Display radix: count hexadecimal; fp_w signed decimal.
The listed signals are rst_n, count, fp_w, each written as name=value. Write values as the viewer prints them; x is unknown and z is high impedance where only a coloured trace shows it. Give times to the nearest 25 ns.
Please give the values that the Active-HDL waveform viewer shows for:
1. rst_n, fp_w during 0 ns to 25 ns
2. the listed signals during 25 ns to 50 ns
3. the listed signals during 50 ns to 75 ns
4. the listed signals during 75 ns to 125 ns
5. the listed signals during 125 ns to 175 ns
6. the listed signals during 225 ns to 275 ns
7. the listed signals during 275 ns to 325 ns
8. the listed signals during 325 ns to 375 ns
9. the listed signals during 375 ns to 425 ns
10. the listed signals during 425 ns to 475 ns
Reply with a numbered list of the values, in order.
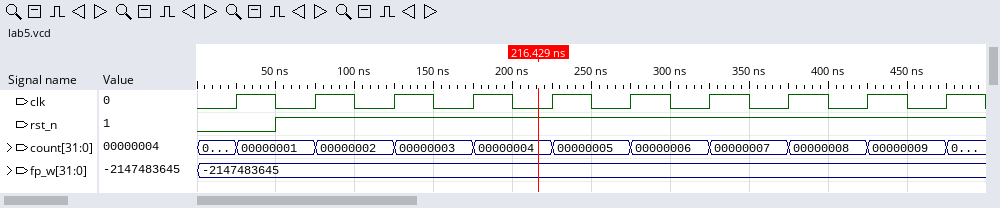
1. rst_n=0, fp_w=-2147483645
2. rst_n=0, count=00000001, fp_w=-2147483645
3. rst_n=1, count=00000001, fp_w=-2147483645
4. rst_n=1, count=00000002, fp_w=-2147483645
5. rst_n=1, count=00000003, fp_w=-2147483645
6. rst_n=1, count=00000005, fp_w=-2147483645
7. rst_n=1, count=00000006, fp_w=-2147483645
8. rst_n=1, count=00000007, fp_w=-2147483645
9. rst_n=1, count=00000008, fp_w=-2147483645
10. rst_n=1, count=00000009, fp_w=-2147483645
